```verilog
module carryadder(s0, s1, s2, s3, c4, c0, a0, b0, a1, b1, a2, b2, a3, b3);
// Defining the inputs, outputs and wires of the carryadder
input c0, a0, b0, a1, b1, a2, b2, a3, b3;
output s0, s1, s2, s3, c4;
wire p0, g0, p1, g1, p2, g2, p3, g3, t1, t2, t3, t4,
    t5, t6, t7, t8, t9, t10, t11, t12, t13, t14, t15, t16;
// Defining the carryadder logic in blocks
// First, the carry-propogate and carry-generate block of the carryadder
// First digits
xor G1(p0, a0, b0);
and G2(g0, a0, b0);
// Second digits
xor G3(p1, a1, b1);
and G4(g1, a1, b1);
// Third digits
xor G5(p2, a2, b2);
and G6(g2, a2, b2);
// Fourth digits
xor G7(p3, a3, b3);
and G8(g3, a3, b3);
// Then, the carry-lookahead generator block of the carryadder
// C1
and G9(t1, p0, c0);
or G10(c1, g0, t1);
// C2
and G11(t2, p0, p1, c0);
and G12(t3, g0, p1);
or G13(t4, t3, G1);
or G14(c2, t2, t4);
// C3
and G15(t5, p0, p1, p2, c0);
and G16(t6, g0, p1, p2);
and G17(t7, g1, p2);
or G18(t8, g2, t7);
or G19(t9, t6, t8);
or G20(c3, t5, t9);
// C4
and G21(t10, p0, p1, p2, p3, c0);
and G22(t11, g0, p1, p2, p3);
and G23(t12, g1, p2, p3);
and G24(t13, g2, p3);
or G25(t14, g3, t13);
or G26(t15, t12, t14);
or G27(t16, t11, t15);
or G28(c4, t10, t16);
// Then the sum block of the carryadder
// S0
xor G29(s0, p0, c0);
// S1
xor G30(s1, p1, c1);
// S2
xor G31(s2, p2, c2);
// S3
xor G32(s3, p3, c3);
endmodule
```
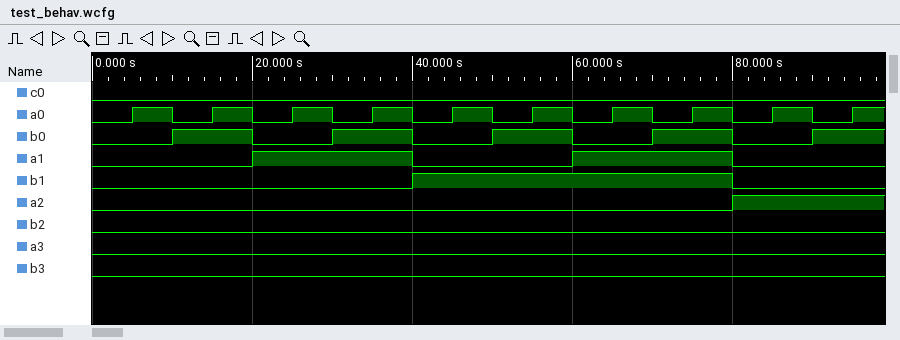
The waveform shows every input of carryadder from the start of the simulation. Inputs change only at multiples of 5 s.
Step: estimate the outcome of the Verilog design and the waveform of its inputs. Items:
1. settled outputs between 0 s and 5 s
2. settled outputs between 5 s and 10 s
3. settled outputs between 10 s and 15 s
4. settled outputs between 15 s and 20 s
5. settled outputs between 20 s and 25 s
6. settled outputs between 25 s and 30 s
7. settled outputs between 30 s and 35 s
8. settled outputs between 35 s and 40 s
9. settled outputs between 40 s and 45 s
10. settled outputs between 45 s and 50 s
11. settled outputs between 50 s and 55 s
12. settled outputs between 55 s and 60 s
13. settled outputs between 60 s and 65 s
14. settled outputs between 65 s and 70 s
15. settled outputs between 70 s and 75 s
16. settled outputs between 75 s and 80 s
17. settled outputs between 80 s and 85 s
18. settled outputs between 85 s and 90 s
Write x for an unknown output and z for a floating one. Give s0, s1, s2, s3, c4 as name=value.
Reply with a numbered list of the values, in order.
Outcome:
1. s0=0, s1=0, s2=x, s3=0, c4=0
2. s0=1, s1=0, s2=x, s3=0, c4=0
3. s0=1, s1=0, s2=x, s3=0, c4=0
4. s0=0, s1=1, s2=x, s3=0, c4=0
5. s0=0, s1=1, s2=x, s3=0, c4=0
6. s0=1, s1=1, s2=x, s3=0, c4=0
7. s0=1, s1=1, s2=x, s3=0, c4=0
8. s0=0, s1=0, s2=1, s3=0, c4=0
9. s0=0, s1=1, s2=x, s3=0, c4=0
10. s0=1, s1=1, s2=x, s3=0, c4=0
11. s0=1, s1=1, s2=x, s3=0, c4=0
12. s0=0, s1=0, s2=1, s3=0, c4=0
13. s0=0, s1=0, s2=x, s3=0, c4=0
14. s0=1, s1=0, s2=x, s3=0, c4=0
15. s0=1, s1=0, s2=x, s3=0, c4=0
16. s0=0, s1=1, s2=x, s3=0, c4=0
17. s0=0, s1=0, s2=x, s3=0, c4=0
18. s0=1, s1=0, s2=x, s3=0, c4=0
